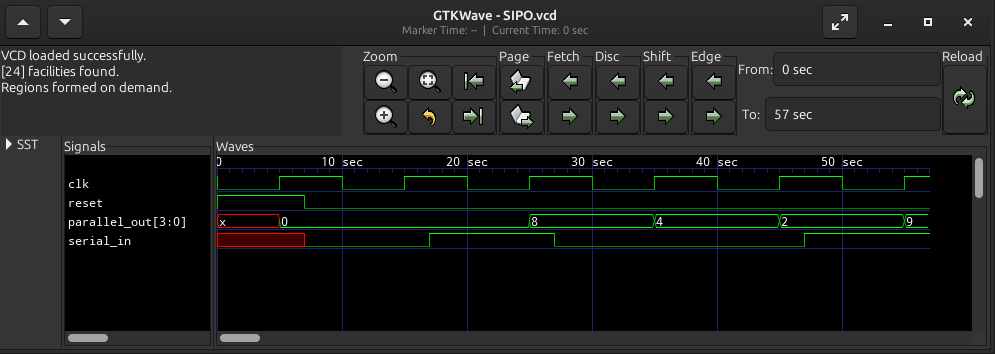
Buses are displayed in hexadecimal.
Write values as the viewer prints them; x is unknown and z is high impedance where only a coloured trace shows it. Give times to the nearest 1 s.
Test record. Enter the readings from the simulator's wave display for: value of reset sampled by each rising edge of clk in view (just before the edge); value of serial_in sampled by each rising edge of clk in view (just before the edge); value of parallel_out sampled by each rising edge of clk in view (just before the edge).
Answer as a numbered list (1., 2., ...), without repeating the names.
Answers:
1. 1 0 0 0 0 0
2. x 0 1 0 0 1
3. x, 0, 0, 8, 4, 2
